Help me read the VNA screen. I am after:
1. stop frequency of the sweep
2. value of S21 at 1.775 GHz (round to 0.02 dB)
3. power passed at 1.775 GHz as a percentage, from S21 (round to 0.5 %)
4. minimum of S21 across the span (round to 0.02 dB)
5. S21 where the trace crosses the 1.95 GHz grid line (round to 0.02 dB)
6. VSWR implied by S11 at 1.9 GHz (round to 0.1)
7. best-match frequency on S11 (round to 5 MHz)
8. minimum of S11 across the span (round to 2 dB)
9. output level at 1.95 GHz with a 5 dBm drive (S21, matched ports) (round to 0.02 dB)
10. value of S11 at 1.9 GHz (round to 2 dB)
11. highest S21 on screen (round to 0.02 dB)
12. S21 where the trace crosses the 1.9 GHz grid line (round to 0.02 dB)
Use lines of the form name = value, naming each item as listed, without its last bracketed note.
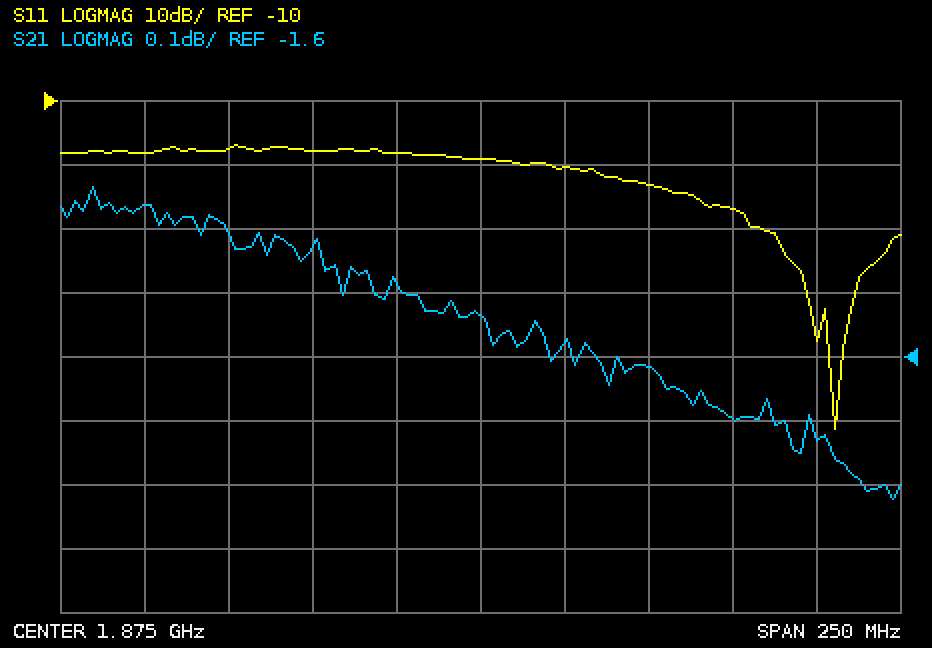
stop frequency of the sweep = 2 GHz
value of S21 at 1.775 GHz = -1.36 dB
power passed at 1.775 GHz as a percentage, from S21 = 73.0 %
minimum of S21 across the span = -1.82 dB
S21 where the trace crosses the 1.95 GHz grid line = -1.70 dB
VSWR implied by S11 at 1.9 GHz = 1.2
best-match frequency on S11 = 1.980 GHz
minimum of S11 across the span = -62 dB
output level at 1.95 GHz with a 5 dBm drive (S21, matched ports) = 3.30 dBm
value of S11 at 1.9 GHz = -20 dB
highest S21 on screen = -1.34 dB
S21 where the trace crosses the 1.9 GHz grid line = -1.58 dB
